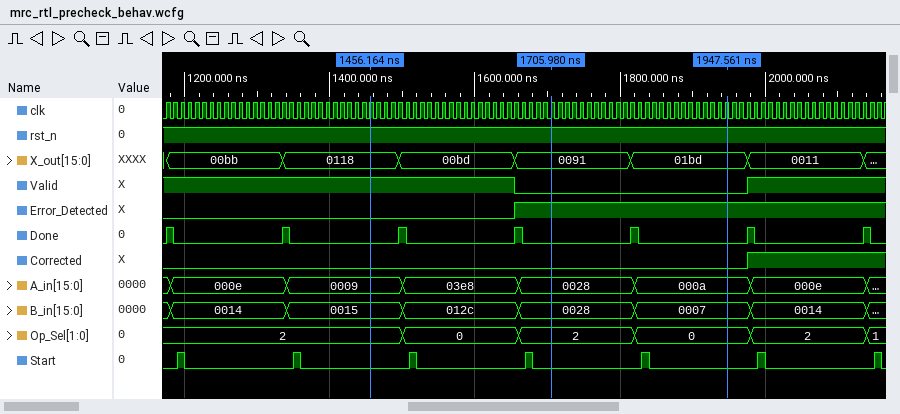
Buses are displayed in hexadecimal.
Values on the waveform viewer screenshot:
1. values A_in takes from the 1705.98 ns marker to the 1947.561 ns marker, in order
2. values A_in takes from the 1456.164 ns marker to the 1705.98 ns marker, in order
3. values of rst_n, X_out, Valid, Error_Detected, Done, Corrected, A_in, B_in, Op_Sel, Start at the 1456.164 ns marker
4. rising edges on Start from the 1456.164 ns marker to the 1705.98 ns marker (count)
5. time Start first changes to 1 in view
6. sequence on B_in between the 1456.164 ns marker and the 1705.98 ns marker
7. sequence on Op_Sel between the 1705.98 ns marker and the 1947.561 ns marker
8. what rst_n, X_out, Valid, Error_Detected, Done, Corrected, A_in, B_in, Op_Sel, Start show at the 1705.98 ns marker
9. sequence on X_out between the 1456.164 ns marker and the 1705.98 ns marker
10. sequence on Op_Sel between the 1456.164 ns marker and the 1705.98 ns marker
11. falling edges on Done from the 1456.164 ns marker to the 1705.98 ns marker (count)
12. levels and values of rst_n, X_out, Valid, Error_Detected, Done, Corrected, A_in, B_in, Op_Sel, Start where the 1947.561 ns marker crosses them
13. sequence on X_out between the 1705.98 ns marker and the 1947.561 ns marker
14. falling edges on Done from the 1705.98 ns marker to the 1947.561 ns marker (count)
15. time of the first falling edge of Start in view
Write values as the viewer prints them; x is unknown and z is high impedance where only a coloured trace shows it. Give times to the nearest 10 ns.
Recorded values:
0028, 000a
0009, 03e8, 0028
rst_n=1, X_out=0118, Valid=1, Error_Detected=0, Done=0, Corrected=0, A_in=0009, B_in=0015, Op_Sel=2, Start=0
2
1190 ns
0015, 012c, 0028
2, 0
rst_n=1, X_out=0091, Valid=0, Error_Detected=1, Done=0, Corrected=0, A_in=0028, B_in=0028, Op_Sel=2, Start=0
0118, 00bd, 0091
2, 0, 2
2
rst_n=1, X_out=01bd, Valid=0, Error_Detected=1, Done=0, Corrected=0, A_in=000a, B_in=0007, Op_Sel=0, Start=0
0091, 01bd
1
1200 ns
